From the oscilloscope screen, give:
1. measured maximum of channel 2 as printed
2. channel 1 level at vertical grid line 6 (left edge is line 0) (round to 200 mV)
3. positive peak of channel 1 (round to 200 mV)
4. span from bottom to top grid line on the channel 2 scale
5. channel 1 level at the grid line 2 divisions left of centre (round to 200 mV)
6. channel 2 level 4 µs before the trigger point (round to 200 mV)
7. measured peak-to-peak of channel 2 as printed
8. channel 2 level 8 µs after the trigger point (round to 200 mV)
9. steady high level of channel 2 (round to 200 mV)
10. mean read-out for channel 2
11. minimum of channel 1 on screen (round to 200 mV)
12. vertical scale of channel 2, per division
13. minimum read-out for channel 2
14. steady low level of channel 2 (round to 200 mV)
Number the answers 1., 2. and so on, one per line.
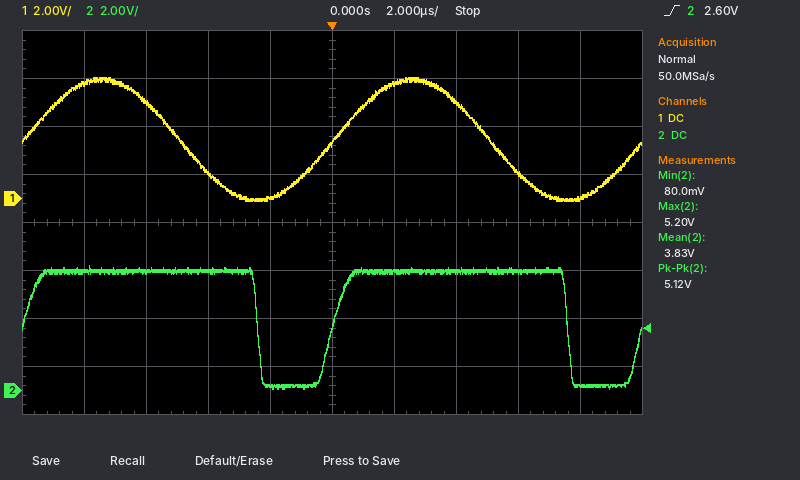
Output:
1. 5.20 V
2. 4.8 V
3. 5.0 V
4. 16 V
5. 1.0 V
6. 5.0 V
7. 5.12 V
8. 200 mV
9. 5.0 V
10. 3.83 V
11. 0.0 V
12. 2 V
13. 80.0 mV
14. 200 mV
